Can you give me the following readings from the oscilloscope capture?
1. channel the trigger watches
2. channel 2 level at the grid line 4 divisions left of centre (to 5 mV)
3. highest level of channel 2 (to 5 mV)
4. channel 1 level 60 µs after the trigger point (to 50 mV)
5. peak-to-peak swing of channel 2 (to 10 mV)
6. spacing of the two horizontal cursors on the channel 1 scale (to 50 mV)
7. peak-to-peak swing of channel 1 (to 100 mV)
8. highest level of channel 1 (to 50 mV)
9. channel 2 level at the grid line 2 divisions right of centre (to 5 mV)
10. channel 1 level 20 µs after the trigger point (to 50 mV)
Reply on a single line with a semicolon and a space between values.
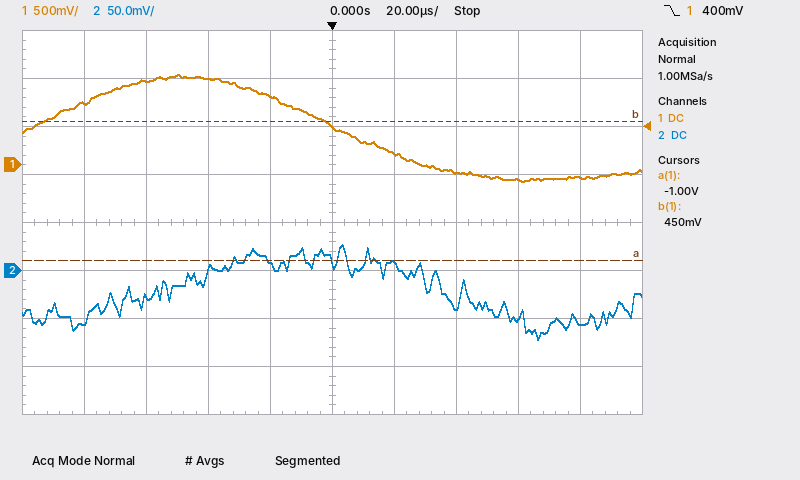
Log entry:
channel 1; -55 mV; 25 mV; -150 mV; 100 mV; 1.45 V; 1.10 V; 950 mV; -35 mV; 100 mV
